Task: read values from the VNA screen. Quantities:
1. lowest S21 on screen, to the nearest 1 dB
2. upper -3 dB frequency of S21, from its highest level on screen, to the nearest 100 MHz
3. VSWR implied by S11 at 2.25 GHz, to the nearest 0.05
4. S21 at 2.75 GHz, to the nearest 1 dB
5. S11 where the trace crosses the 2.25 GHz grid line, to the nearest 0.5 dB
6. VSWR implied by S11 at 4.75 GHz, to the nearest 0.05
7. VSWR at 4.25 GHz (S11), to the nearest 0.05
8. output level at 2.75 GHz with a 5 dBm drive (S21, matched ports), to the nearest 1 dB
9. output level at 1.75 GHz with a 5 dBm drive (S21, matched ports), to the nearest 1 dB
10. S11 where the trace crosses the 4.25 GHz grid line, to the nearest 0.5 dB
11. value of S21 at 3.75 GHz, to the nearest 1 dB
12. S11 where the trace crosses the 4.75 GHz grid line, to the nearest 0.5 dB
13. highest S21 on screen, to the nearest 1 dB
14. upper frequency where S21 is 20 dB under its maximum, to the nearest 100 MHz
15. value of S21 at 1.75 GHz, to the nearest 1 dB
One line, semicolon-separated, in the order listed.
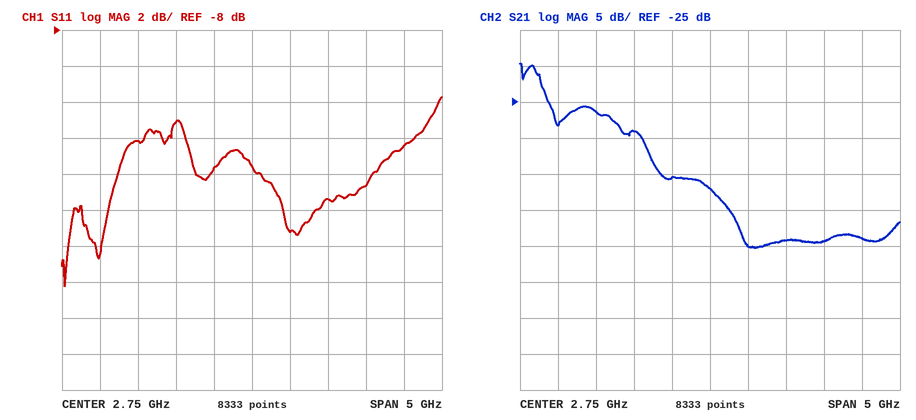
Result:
-45 dB; 500 MHz; 1.40; -37 dB; -15.5 dB; 1.45; 1.35; -32 dBm; -24 dBm; -16.5 dB; -44 dB; -14.5 dB; -20 dB; 3.0 GHz; -29 dB
